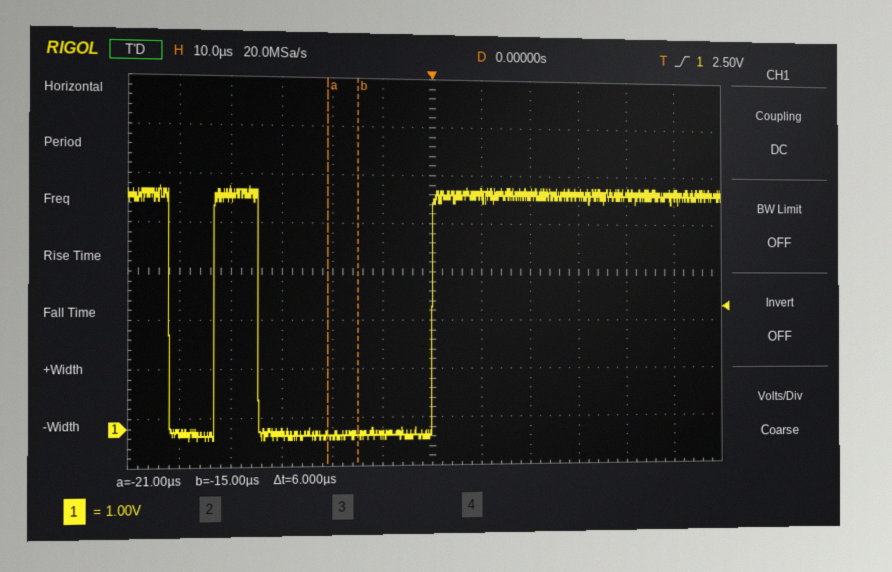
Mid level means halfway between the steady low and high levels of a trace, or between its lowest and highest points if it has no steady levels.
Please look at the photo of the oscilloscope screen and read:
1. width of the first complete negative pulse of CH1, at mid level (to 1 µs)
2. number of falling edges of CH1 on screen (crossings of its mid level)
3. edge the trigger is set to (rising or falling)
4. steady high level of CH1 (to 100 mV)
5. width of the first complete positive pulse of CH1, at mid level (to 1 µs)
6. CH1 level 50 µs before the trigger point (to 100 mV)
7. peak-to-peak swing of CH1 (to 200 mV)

9 µs
2
rising
4.8 V
9 µs
-100 mV
5.2 V
